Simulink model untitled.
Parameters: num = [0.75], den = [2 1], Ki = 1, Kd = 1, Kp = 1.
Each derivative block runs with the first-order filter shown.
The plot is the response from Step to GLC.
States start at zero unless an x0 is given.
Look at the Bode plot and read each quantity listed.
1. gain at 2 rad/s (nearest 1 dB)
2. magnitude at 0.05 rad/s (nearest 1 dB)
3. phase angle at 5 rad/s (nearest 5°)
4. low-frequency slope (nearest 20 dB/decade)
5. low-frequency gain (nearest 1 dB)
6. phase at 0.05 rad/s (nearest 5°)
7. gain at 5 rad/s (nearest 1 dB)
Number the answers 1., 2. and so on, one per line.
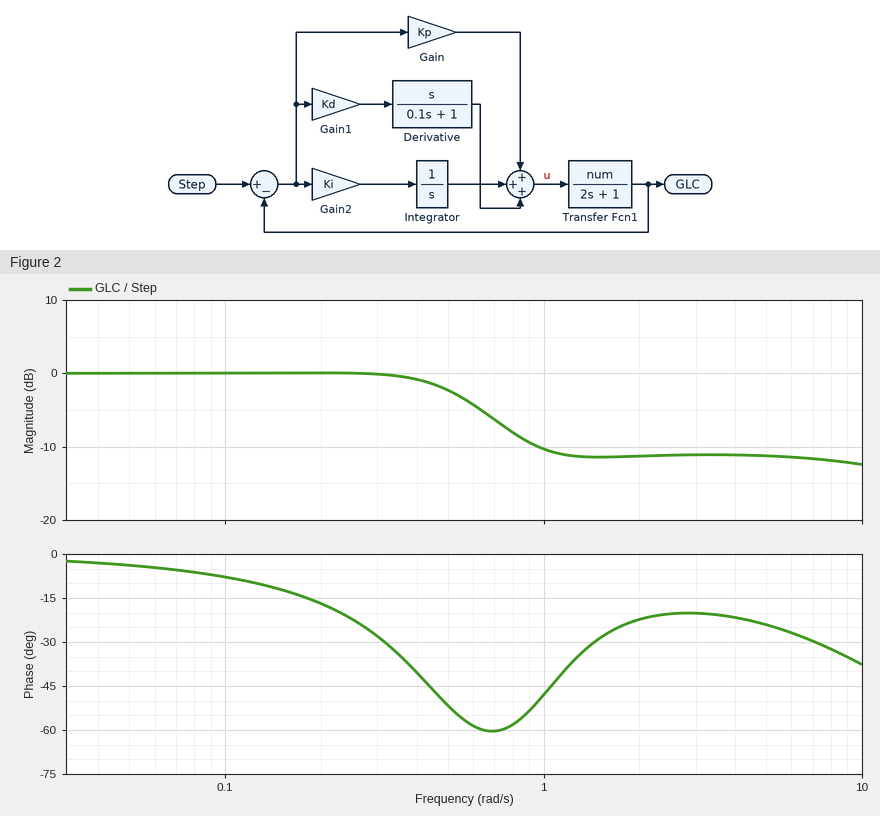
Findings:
1. -11 dB
2. 0 dB
3. -25°
4. 0 dB/decade
5. 0 dB
6. -5°
7. -11 dB
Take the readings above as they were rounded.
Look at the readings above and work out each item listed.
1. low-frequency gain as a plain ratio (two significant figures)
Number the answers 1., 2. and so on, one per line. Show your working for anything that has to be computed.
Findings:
1. 10^(0 / 20) = 1.0
